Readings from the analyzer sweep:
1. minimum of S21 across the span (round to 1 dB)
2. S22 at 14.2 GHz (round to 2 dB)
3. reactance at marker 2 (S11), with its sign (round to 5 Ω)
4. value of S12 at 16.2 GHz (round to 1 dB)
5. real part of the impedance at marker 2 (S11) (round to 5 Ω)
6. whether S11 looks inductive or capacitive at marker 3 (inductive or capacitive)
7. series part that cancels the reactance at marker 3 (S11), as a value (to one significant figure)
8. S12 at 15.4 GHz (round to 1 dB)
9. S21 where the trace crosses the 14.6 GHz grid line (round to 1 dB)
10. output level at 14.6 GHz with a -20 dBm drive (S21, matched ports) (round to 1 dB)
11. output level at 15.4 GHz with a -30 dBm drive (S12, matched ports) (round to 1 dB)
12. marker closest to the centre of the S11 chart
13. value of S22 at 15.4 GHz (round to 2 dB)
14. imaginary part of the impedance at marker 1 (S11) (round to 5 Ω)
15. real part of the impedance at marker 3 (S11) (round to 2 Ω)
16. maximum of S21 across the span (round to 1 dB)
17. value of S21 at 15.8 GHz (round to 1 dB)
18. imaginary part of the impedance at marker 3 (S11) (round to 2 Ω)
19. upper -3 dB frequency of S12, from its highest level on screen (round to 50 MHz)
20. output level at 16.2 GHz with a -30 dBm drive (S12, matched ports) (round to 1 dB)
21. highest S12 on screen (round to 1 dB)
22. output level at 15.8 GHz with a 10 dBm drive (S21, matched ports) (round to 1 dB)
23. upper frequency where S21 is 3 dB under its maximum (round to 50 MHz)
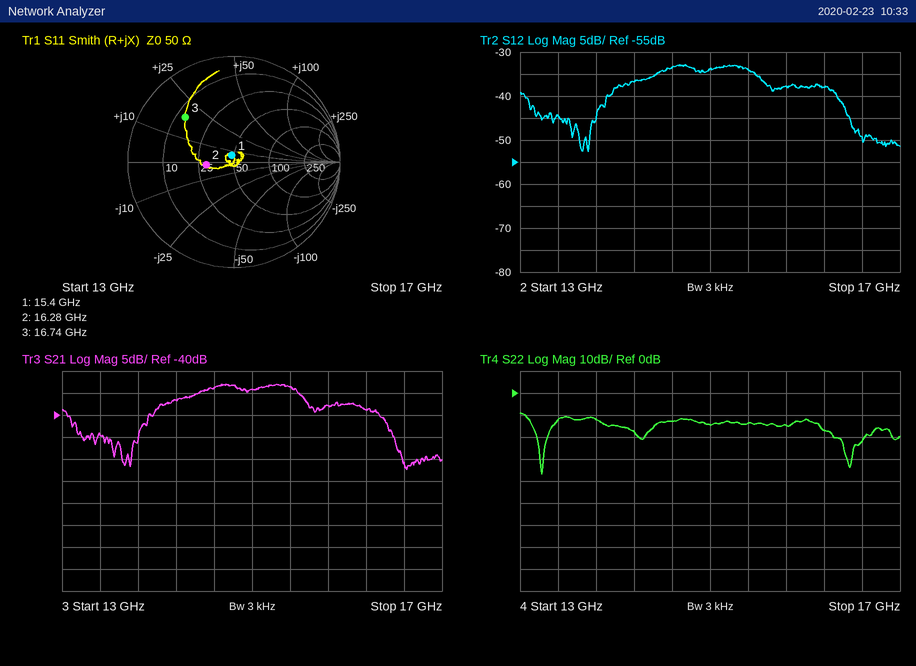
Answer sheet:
-52 dB
-18 dB
0 Ω
-38 dB
30 Ω
inductive
500 fF
-34 dB
-34 dB
-54 dBm
-64 dBm
marker 1
-14 dB
+5 Ω
14 Ω
-33 dB
-38 dB
+18 Ω
15.55 GHz
-68 dBm
-33 dB
-28 dBm
15.55 GHz
